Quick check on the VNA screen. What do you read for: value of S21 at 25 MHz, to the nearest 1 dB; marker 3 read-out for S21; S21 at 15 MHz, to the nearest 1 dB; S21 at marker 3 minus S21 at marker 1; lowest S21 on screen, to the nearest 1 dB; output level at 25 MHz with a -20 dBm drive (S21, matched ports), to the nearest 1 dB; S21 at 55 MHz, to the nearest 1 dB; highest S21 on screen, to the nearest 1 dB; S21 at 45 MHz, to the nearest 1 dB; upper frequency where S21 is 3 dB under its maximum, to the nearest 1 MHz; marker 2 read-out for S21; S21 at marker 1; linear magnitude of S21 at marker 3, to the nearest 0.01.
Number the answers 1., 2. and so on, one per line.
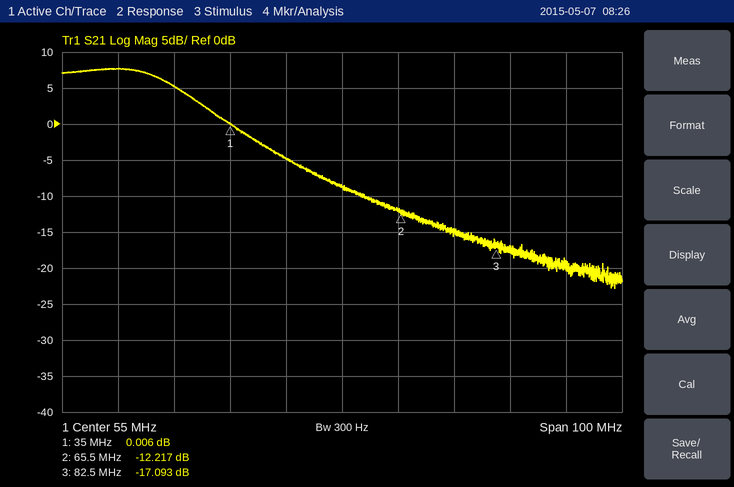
1. 5 dB
2. -17.093 dB
3. 8 dB
4. -17.099 dB
5. -23 dB
6. -15 dBm
7. -9 dB
8. 8 dB
9. -5 dB
10. 26 MHz
11. -12.217 dB
12. 0.006 dB
13. 0.14
